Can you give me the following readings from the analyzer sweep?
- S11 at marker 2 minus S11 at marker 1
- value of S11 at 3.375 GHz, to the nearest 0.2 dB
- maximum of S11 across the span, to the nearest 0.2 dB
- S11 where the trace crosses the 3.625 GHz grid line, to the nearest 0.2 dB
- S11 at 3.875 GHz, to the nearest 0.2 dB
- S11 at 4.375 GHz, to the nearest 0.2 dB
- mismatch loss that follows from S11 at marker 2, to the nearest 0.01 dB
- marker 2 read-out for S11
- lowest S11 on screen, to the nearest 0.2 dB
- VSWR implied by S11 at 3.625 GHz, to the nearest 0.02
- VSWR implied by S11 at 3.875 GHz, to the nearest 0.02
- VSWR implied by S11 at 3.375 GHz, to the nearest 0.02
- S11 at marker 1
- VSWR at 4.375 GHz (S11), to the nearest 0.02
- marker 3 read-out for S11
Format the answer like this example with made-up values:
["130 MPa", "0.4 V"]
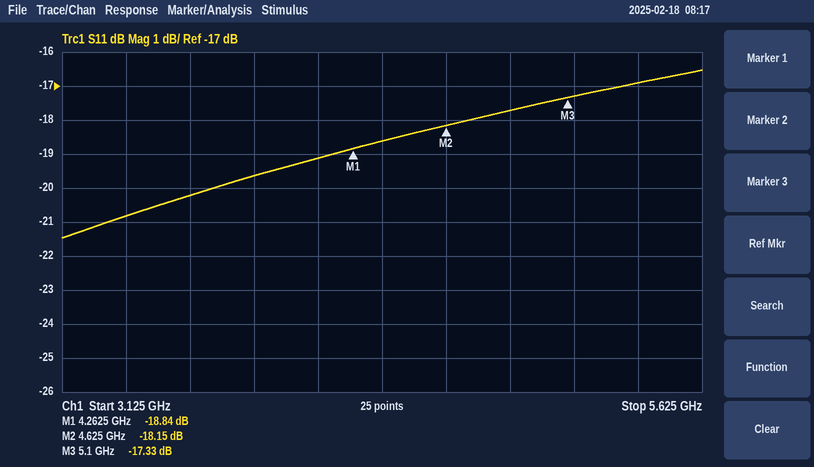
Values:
["0.69 dB", "-20.8 dB", "-16.6 dB", "-20.2 dB", "-19.6 dB", "-18.6 dB", "0.07 dB", "-18.15 dB", "-21.4 dB", "1.22", "1.24", "1.20", "-18.84 dB", "1.26", "-17.33 dB"]
